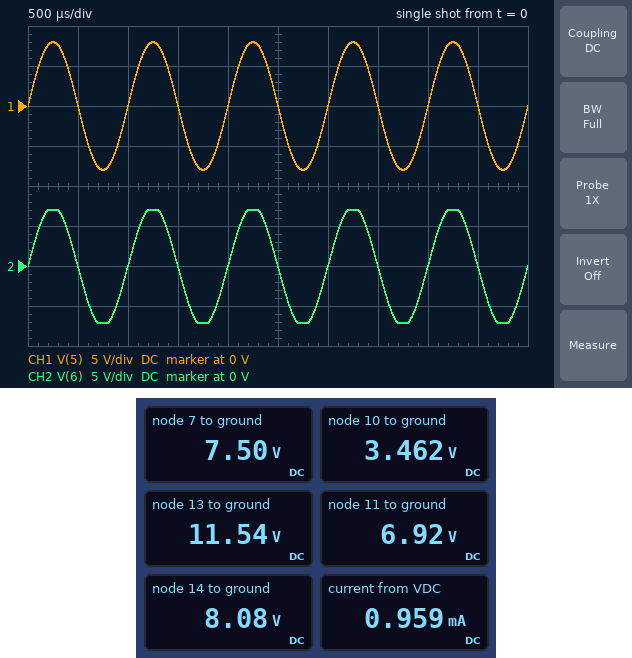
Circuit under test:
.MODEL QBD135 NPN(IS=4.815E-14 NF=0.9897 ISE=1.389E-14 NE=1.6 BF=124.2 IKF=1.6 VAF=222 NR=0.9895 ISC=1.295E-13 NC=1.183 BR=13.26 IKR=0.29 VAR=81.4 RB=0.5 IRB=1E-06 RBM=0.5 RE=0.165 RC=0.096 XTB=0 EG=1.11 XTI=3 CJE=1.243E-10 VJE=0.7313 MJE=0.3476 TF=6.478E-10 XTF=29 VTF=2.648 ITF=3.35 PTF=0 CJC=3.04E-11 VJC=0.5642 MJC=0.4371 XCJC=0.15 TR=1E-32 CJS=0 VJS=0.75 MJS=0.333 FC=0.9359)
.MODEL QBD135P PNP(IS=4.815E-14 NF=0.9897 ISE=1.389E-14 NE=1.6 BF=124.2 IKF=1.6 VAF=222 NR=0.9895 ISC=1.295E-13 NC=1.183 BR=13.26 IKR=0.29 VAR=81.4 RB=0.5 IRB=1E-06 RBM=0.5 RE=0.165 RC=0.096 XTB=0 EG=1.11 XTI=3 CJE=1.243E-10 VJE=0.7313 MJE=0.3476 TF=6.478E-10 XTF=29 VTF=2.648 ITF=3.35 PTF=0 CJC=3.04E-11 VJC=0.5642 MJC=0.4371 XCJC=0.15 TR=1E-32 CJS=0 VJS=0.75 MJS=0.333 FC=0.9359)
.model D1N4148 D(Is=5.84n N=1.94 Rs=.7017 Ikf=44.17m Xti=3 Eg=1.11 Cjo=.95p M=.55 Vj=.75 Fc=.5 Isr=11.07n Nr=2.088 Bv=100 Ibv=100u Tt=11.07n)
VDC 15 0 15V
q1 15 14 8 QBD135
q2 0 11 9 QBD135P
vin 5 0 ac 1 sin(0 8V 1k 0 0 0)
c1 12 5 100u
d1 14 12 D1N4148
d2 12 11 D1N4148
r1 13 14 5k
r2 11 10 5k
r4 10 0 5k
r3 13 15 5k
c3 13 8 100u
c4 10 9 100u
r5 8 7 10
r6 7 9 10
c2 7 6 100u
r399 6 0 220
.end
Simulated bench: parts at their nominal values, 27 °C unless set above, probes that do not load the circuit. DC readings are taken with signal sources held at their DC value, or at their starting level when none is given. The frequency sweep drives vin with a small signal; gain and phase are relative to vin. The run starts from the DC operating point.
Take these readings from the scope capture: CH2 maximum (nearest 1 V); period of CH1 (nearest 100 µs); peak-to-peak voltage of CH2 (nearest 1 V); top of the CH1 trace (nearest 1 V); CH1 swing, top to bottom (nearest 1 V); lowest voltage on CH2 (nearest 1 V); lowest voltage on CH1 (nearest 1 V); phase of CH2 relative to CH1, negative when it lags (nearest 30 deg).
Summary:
7 V
1.0 ms
14 V
8 V
16 V
-7 V
-8 V
0 deg
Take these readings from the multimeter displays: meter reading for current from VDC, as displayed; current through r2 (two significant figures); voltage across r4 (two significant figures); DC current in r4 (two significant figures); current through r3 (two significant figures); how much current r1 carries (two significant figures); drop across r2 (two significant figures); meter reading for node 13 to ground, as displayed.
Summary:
0.959 mA
690 µA
3.5 V
690 µA
690 µA
690 µA
3.5 V
11.54 V
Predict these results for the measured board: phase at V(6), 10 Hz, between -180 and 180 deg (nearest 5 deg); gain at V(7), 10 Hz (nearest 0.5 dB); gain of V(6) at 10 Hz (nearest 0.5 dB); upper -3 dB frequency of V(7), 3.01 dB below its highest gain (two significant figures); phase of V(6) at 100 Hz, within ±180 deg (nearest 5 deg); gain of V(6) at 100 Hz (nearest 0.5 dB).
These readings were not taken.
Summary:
30 deg
-1.5 dB
-3.5 dB
8.2 Hz
5 deg
-2.0 dB
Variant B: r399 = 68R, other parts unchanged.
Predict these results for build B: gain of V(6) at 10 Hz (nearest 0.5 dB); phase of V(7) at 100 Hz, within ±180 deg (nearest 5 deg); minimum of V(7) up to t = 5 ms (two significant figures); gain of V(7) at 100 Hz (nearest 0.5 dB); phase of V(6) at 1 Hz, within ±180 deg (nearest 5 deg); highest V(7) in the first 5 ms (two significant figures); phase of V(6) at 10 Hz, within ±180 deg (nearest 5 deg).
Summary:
-9.5 dB
-5 deg
2.3 V
-5.0 dB
90 deg
13 V
55 deg
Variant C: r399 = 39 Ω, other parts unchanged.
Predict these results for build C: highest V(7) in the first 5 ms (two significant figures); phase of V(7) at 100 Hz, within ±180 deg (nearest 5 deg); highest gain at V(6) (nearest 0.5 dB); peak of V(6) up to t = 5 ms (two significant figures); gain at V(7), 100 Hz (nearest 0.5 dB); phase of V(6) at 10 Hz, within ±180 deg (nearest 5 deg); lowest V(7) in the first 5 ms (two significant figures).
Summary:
11 V
-10 deg
-7.5 dB
3.1 V
-7.0 dB
60 deg
4.5 V
